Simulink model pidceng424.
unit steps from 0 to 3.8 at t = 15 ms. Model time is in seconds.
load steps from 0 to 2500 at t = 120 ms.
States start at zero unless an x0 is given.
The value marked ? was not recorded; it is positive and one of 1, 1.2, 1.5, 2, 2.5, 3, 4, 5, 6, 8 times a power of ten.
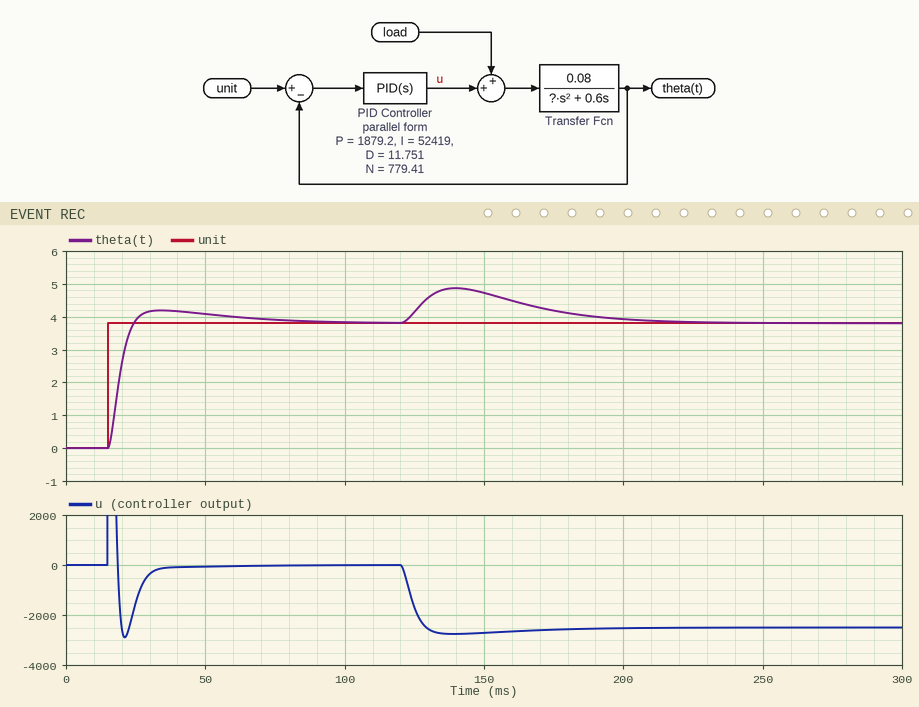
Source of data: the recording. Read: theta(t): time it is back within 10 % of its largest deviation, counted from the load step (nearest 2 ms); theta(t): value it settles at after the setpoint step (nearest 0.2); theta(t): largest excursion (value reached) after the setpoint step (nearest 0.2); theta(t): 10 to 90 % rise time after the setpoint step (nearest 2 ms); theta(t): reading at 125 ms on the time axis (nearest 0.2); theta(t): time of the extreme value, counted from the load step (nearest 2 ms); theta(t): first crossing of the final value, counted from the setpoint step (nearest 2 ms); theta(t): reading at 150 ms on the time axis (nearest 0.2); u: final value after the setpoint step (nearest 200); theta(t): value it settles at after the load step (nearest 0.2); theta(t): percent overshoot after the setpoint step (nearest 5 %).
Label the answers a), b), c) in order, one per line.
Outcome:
a) 84 ms
b) 3.8
c) 4.2
d) 6 ms
e) 4.2
f) 20 ms
g) 10 ms
h) 4.8
i) 0
j) 3.8
k) 10 %
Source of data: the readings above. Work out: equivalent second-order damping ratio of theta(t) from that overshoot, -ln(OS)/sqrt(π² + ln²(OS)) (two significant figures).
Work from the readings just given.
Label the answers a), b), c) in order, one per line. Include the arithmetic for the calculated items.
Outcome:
a) ln(0.1) = -2.303; 2.303 / sqrt(9.870 + 5.302) = 0.59
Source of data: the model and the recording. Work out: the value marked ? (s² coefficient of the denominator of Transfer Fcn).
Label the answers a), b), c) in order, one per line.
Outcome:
a) 0.005
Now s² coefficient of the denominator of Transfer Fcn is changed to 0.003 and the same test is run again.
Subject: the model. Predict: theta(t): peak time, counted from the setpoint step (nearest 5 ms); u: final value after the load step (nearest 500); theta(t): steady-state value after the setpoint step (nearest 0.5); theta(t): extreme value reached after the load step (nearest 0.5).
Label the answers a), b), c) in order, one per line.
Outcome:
a) 30 ms
b) -2500
c) 4.0
d) 5.0
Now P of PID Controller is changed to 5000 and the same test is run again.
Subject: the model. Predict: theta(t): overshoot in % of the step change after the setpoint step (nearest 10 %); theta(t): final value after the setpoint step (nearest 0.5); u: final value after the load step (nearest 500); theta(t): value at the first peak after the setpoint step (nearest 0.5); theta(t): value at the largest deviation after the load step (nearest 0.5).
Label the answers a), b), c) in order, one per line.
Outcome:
a) 30 %
b) 4.0
c) -2500
d) 5.0
e) 4.5
